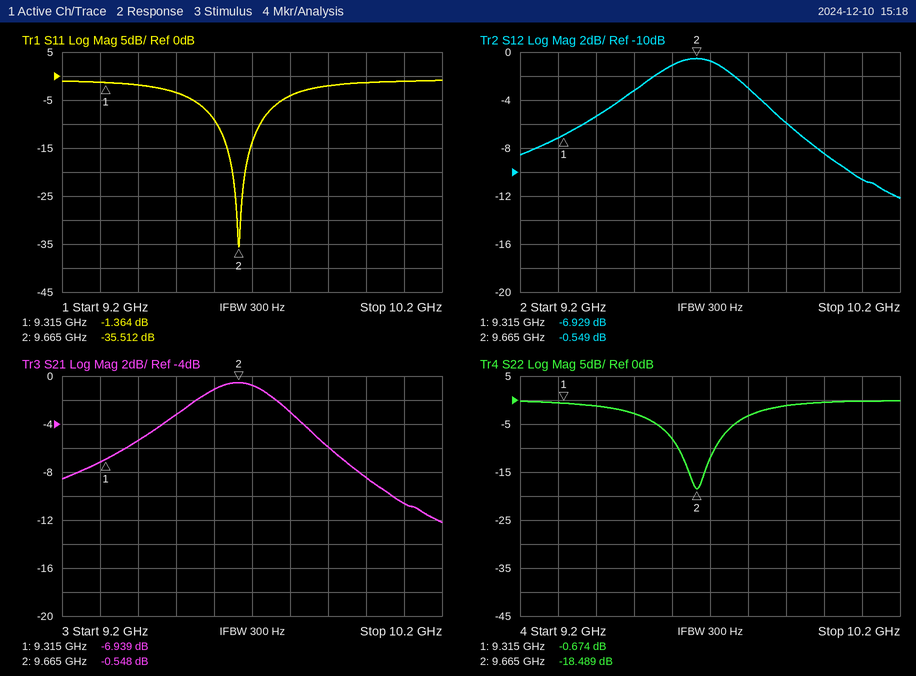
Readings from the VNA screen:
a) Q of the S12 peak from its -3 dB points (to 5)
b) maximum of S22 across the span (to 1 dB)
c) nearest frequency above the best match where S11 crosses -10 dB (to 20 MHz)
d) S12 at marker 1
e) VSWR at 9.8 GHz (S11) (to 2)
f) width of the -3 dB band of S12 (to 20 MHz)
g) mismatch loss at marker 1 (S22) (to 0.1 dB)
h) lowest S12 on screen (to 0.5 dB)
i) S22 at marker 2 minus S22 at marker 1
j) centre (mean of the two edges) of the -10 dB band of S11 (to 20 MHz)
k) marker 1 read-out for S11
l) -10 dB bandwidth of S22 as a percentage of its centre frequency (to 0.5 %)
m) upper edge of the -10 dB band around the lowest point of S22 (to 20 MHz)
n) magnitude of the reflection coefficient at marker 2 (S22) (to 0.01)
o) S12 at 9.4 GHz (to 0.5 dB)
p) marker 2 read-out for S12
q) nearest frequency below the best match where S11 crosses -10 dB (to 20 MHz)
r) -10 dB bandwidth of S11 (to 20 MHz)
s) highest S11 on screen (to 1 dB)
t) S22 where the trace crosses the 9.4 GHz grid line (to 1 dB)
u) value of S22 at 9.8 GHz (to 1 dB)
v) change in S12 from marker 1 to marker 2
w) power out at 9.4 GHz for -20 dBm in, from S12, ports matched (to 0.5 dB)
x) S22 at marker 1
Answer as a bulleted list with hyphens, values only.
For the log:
- 30
- 0 dB
- 9.72 GHz
- -6.929 dB
- 4
- 340 MHz
- 8.4 dB
- -12.0 dB
- -17.815 dB
- 9.66 GHz
- -1.364 dB
- 1.0 %
- 9.72 GHz
- 0.12
- -5.5 dB
- -0.549 dB
- 9.60 GHz
- 120 MHz
- -1 dB
- -1 dB
- -3 dB
- 6.380 dB
- -25.5 dBm
- -0.674 dB
